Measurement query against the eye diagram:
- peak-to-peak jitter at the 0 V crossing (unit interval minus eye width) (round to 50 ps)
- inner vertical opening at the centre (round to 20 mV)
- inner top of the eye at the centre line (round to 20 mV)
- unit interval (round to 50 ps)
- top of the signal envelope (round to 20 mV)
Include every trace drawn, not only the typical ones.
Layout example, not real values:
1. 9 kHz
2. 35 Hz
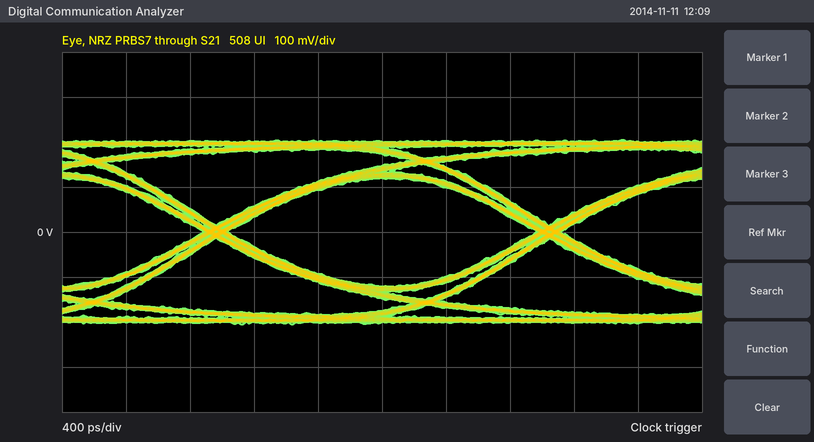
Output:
1. 150 ps
2. 240 mV
3. 120 mV
4. 2.10 ns
5. 200 mV
